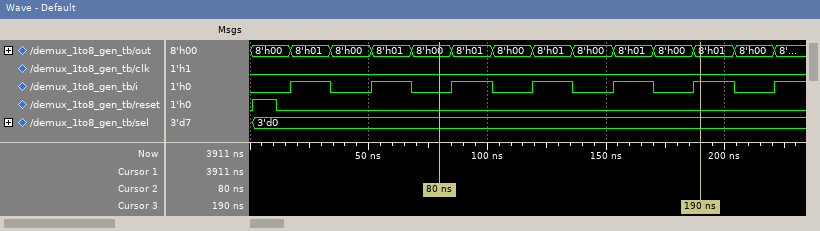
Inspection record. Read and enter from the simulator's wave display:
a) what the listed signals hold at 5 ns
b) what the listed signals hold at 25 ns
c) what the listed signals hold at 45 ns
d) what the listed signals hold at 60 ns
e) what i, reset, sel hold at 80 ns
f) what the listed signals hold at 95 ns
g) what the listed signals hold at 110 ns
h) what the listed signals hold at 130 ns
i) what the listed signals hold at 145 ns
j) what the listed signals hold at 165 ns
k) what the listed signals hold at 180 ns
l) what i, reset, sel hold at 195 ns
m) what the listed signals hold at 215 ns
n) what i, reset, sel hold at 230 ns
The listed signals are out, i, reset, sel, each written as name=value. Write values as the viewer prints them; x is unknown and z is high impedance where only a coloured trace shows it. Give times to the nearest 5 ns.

out=8'h00, i=0, reset=1, sel=3'd0
out=8'h01, i=1, reset=0, sel=3'd0
out=8'h00, i=0, reset=0, sel=3'd0
out=8'h01, i=1, reset=0, sel=3'd0
i=0, reset=0, sel=3'd0
out=8'h01, i=1, reset=0, sel=3'd0
out=8'h00, i=0, reset=0, sel=3'd0
out=8'h01, i=1, reset=0, sel=3'd0
out=8'h00, i=0, reset=0, sel=3'd0
out=8'h01, i=1, reset=0, sel=3'd0
out=8'h00, i=0, reset=0, sel=3'd0
i=1, reset=0, sel=3'd0
out=8'h00, i=0, reset=0, sel=3'd0
i=1, reset=0, sel=3'd0
